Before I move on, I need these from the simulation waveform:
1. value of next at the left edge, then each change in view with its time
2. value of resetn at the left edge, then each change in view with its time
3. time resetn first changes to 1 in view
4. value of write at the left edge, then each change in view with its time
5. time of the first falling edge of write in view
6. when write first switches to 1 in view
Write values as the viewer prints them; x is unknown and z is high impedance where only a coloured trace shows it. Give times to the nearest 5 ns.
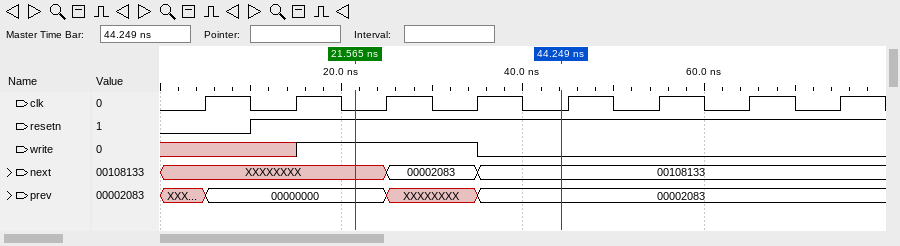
XXXXXXXX, 00002083 at 25 ns, 00108133 at 35 ns
0, 1 at 10 ns
10 ns
x, 1 at 15 ns, 0 at 35 ns
35 ns
15 ns
